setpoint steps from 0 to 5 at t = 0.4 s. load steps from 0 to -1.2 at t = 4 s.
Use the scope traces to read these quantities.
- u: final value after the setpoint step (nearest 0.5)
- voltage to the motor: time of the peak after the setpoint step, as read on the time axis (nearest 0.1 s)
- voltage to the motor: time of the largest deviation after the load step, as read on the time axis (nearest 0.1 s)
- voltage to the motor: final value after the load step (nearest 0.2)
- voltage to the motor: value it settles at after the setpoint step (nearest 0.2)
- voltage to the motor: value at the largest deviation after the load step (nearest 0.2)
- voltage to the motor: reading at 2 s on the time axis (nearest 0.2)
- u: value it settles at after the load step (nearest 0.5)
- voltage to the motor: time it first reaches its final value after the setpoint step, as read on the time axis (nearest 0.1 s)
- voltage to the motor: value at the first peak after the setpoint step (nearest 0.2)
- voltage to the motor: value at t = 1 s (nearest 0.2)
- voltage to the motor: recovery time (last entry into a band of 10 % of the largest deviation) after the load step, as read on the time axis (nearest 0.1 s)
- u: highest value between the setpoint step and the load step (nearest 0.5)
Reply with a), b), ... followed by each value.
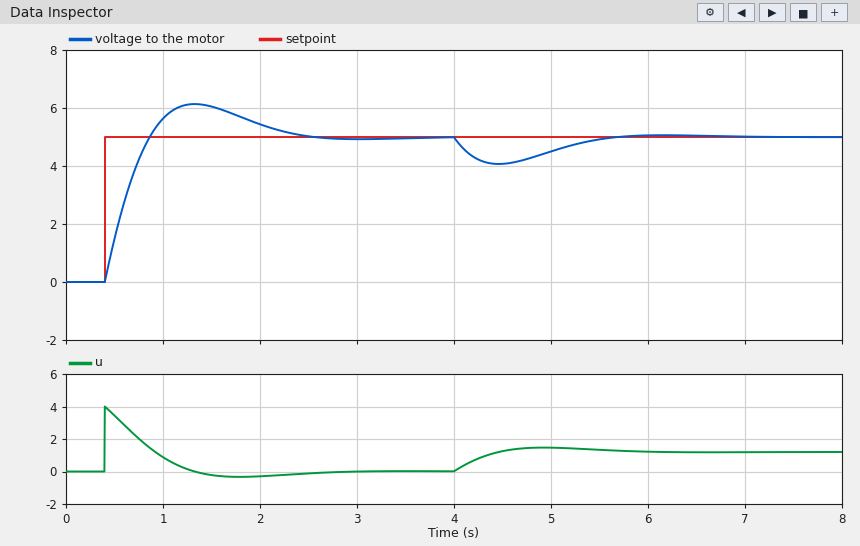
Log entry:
a) 0.0
b) 1.3 s
c) 4.5 s
d) 5.0
e) 5.0
f) 4.0
g) 5.4
h) 1.0
i) 0.9 s
j) 6.2
k) 5.6
l) 5.5 s
m) 4.0
